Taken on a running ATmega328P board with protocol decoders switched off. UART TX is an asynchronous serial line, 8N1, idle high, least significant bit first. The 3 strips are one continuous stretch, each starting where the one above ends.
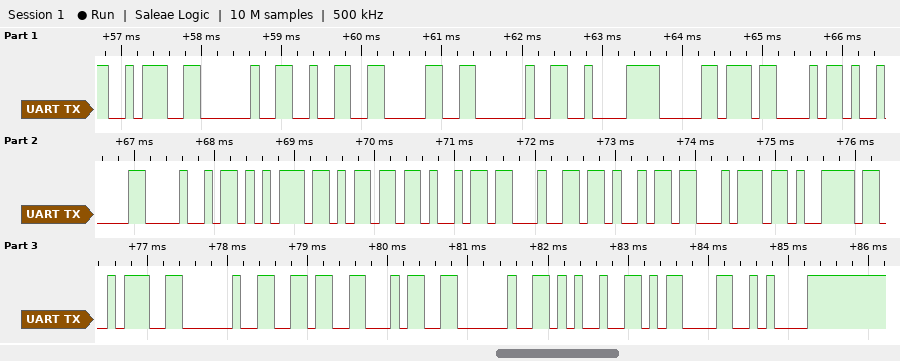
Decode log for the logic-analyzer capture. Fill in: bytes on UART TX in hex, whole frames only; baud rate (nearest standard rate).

3A 20 32 30 20 C2 B0 43 09 48 75 6D 69 64 69 74 79 3A 20 36 34 20 25 0D 0A
9600 baud
